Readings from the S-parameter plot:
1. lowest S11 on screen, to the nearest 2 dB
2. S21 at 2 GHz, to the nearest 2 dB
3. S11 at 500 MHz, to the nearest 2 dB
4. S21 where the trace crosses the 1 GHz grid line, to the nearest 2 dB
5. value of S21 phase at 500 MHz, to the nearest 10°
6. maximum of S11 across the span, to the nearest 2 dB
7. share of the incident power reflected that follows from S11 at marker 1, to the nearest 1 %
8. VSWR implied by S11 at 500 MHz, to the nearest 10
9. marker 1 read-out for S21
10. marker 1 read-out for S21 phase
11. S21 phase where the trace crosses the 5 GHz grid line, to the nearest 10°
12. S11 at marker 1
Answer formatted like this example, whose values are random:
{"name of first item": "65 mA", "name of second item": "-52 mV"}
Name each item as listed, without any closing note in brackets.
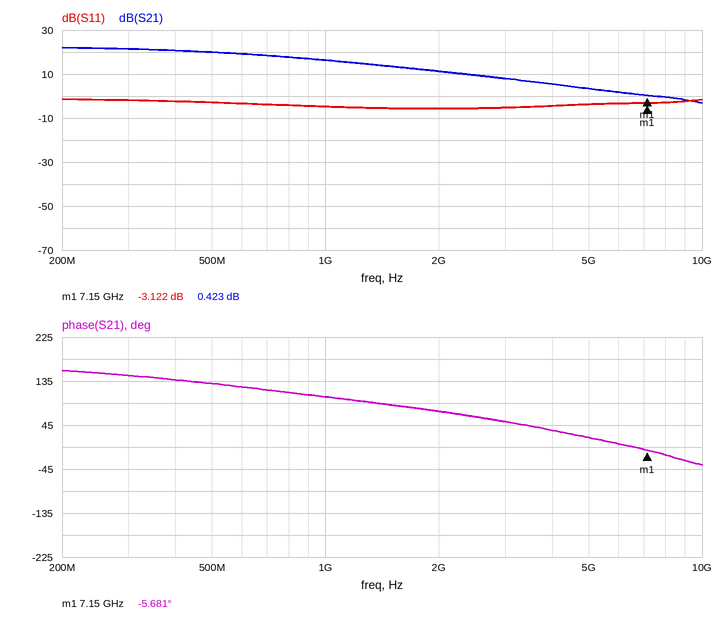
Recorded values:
{"lowest S11 on screen, to the nearest 2 dB": "-6 dB", "S21 at 2 GHz, to the nearest 2 dB": "12 dB", "S11 at 500 MHz, to the nearest 2 dB": "-2 dB", "S21 where the trace crosses the 1 GHz grid line, to the nearest 2 dB": "16 dB", "value of S21 phase at 500 MHz, to the nearest 10°": "130°", "maximum of S11 across the span, to the nearest 2 dB": "-2 dB", "share of the incident power reflected that follows from S11 at marker 1, to the nearest 1 %": "49 %", "VSWR implied by S11 at 500 MHz, to the nearest 10": "10", "marker 1 read-out for S21": "0.423 dB", "marker 1 read-out for S21 phase": "-5.681°", "S21 phase where the trace crosses the 5 GHz grid line, to the nearest 10°": "20°", "S11 at marker 1": "-3.122 dB"}
